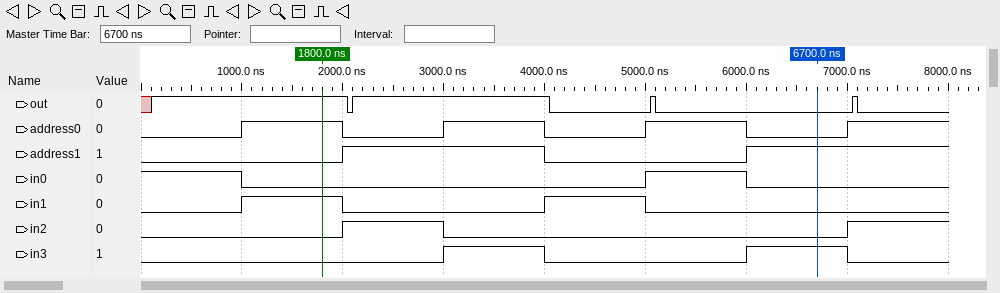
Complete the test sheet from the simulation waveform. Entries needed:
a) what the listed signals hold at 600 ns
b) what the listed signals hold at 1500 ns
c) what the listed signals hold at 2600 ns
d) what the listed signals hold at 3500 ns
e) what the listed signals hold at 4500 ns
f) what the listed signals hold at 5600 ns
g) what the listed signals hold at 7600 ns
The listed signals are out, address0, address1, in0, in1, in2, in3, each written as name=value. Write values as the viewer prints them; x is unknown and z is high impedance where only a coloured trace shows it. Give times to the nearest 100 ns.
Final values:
out=1, address0=0, address1=0, in0=1, in1=0, in2=0, in3=0
out=1, address0=1, address1=0, in0=0, in1=1, in2=0, in3=0
out=1, address0=0, address1=1, in0=0, in1=0, in2=1, in3=0
out=1, address0=1, address1=1, in0=0, in1=0, in2=0, in3=1
out=0, address0=0, address1=0, in0=0, in1=1, in2=0, in3=0
out=0, address0=1, address1=0, in0=1, in1=0, in2=0, in3=0
out=0, address0=1, address1=1, in0=0, in1=0, in2=1, in3=0
